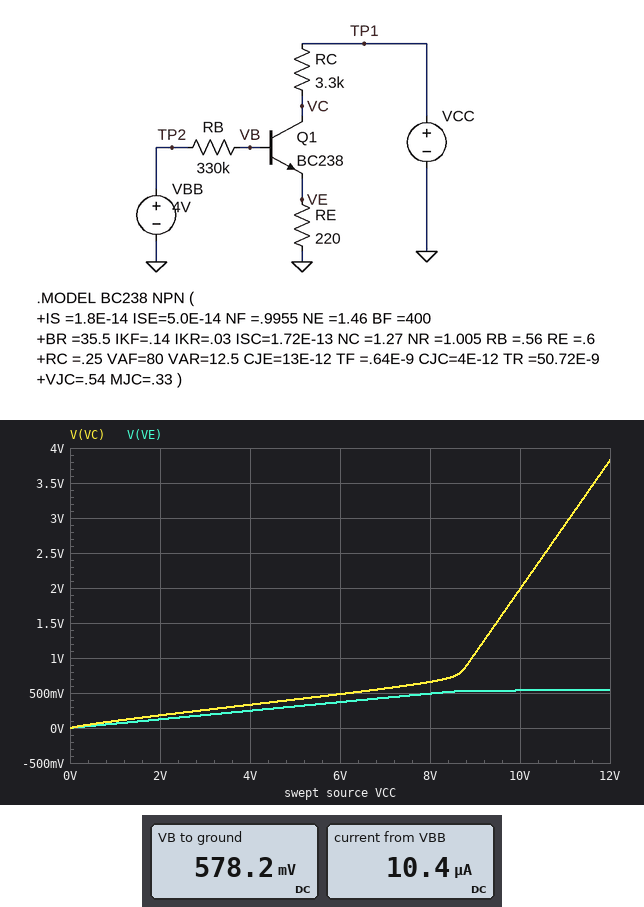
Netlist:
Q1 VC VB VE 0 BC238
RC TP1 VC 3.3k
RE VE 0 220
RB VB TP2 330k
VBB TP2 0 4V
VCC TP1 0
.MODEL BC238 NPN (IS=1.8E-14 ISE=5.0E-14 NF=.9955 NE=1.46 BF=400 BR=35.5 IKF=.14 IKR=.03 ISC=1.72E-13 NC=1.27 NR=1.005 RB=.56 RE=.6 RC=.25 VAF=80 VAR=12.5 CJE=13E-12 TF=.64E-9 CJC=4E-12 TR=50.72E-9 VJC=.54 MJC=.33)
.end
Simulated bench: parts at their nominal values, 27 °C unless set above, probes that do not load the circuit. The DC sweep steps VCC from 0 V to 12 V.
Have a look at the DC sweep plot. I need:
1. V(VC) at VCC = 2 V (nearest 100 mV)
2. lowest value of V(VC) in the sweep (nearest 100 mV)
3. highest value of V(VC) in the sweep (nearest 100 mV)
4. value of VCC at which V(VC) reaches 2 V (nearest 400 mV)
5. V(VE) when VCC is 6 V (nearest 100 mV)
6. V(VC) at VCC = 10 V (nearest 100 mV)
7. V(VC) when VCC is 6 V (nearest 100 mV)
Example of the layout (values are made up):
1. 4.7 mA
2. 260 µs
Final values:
1. 200 mV
2. 0 V
3. 3.8 V
4. 10.0 V
5. 400 mV
6. 2.0 V
7. 500 mV
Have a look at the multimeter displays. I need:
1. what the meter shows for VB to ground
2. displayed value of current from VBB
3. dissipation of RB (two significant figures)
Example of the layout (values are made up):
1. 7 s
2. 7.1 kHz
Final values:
1. 578.2 mV
2. 10.4 µA
3. 35 µW
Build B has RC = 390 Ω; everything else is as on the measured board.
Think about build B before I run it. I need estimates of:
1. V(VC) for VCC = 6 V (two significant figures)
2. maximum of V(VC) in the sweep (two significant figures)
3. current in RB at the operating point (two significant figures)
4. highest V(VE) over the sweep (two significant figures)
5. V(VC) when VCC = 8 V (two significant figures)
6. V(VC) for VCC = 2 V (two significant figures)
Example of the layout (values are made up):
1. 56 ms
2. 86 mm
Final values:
1. 5.0 V
2. 11 V
3. 10 µA
4. 590 mV
5. 7.0 V
6. 1.1 V
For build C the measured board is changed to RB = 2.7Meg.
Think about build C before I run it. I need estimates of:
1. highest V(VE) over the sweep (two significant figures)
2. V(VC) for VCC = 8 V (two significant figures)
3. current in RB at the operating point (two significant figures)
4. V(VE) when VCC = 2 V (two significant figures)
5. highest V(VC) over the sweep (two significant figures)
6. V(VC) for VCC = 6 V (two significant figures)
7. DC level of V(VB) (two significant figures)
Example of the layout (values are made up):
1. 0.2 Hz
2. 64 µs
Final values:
1. 72 mV
2. 7.0 V
3. 1.3 µA
4. 64 mV
5. 11 V
6. 5.0 V
7. 510 mV
